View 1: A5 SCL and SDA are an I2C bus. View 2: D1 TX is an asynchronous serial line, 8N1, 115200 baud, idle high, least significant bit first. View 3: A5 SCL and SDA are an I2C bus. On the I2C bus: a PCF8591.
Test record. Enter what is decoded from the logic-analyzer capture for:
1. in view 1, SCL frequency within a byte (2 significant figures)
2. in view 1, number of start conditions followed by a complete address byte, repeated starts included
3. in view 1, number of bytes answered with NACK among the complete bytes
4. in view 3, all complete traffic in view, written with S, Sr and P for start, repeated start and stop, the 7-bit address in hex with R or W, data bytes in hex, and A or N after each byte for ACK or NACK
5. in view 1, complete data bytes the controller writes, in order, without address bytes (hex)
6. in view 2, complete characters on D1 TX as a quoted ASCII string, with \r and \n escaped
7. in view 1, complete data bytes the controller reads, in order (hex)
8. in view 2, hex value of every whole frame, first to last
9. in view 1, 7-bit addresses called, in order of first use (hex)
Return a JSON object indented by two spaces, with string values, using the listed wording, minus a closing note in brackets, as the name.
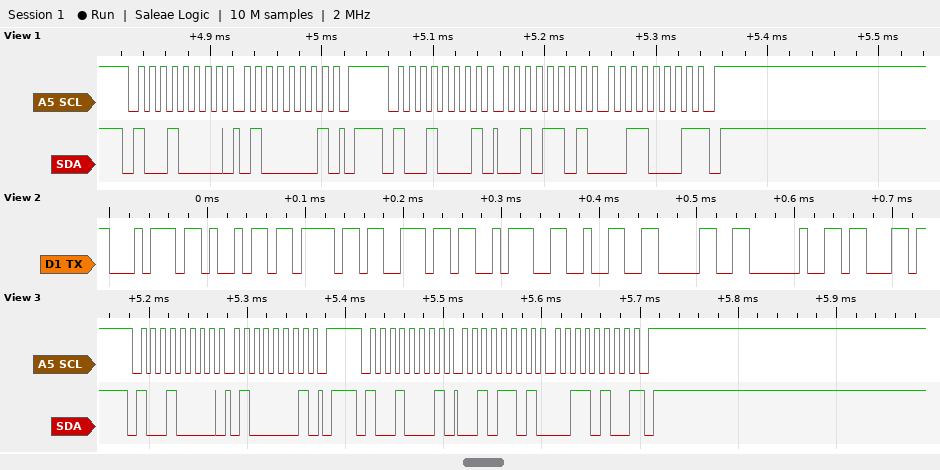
{
  "in view 1, SCL frequency within a byte": "100 kHz",
  "in view 1, number of start conditions followed by a complete address byte, repeated starts included": "2",
  "in view 1, number of bytes answered with NACK among the complete bytes": "1",
  "in view 3, all complete traffic in view, written with S, Sr and P for start, repeated start and stop, the 7-bit address in hex with R or W, data bytes in hex, and A or N after each byte for ACK or NACK": "S 48W A 41 A P S 48R A 2D A 34 N P",
  "in view 1, complete data bytes the controller writes, in order, without address bytes": "41",
  "in view 2, complete characters on D1 TX as a quoted ASCII string, with \\r and \\n escaped": "\"tion:20 c\"",
  "in view 1, complete data bytes the controller reads, in order": "2D 31",
  "in view 2, hex value of every whole frame, first to last": "74 69 6F 6E 3A 32 30 20 63",
  "in view 1, 7-bit addresses called, in order of first use": "0x48"
}
